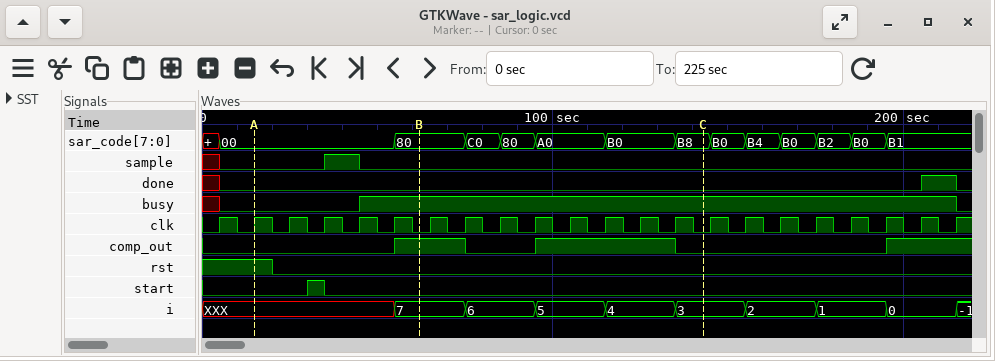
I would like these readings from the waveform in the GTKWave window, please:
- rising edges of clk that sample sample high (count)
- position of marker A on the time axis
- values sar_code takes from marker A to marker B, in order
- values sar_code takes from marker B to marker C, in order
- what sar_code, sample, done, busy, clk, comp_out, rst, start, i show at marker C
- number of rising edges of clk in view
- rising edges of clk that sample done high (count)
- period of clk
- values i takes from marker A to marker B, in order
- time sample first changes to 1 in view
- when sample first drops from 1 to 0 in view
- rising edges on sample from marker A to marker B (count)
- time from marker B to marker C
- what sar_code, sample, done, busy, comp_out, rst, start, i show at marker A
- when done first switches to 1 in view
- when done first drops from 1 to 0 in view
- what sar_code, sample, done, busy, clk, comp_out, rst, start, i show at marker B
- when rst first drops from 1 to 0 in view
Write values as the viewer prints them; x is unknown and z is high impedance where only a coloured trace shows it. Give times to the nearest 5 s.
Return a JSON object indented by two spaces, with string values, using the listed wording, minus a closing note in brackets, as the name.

{
  "rising edges of clk that sample sample high": "1",
  "position of marker A on the time axis": "15 s",
  "values sar_code takes from marker A to marker B, in order": "00, 80",
  "values sar_code takes from marker B to marker C, in order": "80, C0, 80, A0, B0, B8",
  "what sar_code, sample, done, busy, clk, comp_out, rst, start, i show at marker C": "sar_code=B8, sample=0, done=0, busy=1, clk=0, comp_out=0, rst=0, start=0, i=3",
  "number of rising edges of clk in view": "22",
  "rising edges of clk that sample done high": "1",
  "period of clk": "10 s",
  "values i takes from marker A to marker B, in order": "XXX, 7",
  "time sample first changes to 1 in view": "35 s",
  "when sample first drops from 1 to 0 in view": "45 s",
  "rising edges on sample from marker A to marker B": "1",
  "time from marker B to marker C": "80 s",
  "what sar_code, sample, done, busy, comp_out, rst, start, i show at marker A": "sar_code=00, sample=0, done=0, busy=0, comp_out=0, rst=1, start=0, i=XXX",
  "when done first switches to 1 in view": "205 s",
  "when done first drops from 1 to 0 in view": "215 s",
  "what sar_code, sample, done, busy, clk, comp_out, rst, start, i show at marker B": "sar_code=80, sample=0, done=0, busy=1, clk=0, comp_out=1, rst=0, start=0, i=7",
  "when rst first drops from 1 to 0 in view": "20 s"
}
